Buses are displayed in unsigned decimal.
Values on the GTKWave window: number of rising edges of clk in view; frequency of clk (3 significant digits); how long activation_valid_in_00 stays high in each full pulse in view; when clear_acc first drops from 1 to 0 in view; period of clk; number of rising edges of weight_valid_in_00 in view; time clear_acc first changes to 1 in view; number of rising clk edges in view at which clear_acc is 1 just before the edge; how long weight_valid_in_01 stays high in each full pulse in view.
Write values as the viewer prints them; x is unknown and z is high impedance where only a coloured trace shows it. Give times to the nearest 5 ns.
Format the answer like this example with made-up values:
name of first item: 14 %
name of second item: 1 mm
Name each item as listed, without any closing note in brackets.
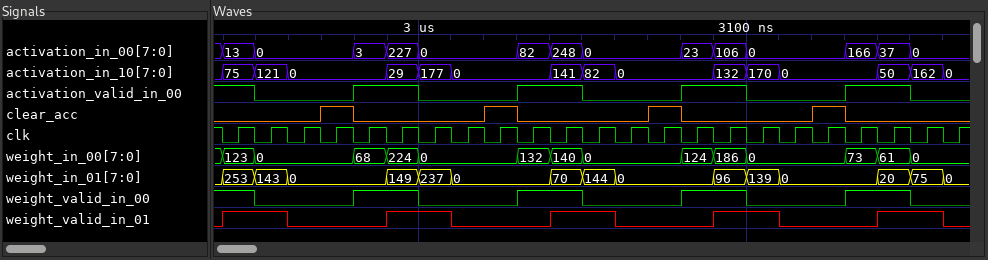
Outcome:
number of rising edges of clk in view: 23
frequency of clk: 100 MHz
how long activation_valid_in_00 stays high in each full pulse in view: 20 ns, 20 ns, 20 ns, 20 ns
when clear_acc first drops from 1 to 0 in view: 2980 ns
period of clk: 10 ns
number of rising edges of weight_valid_in_00 in view: 4
time clear_acc first changes to 1 in view: 2970 ns
number of rising clk edges in view at which clear_acc is 1 just before the edge: 4
how long weight_valid_in_01 stays high in each full pulse in view: 20 ns, 20 ns, 20 ns, 20 ns, 20 ns
